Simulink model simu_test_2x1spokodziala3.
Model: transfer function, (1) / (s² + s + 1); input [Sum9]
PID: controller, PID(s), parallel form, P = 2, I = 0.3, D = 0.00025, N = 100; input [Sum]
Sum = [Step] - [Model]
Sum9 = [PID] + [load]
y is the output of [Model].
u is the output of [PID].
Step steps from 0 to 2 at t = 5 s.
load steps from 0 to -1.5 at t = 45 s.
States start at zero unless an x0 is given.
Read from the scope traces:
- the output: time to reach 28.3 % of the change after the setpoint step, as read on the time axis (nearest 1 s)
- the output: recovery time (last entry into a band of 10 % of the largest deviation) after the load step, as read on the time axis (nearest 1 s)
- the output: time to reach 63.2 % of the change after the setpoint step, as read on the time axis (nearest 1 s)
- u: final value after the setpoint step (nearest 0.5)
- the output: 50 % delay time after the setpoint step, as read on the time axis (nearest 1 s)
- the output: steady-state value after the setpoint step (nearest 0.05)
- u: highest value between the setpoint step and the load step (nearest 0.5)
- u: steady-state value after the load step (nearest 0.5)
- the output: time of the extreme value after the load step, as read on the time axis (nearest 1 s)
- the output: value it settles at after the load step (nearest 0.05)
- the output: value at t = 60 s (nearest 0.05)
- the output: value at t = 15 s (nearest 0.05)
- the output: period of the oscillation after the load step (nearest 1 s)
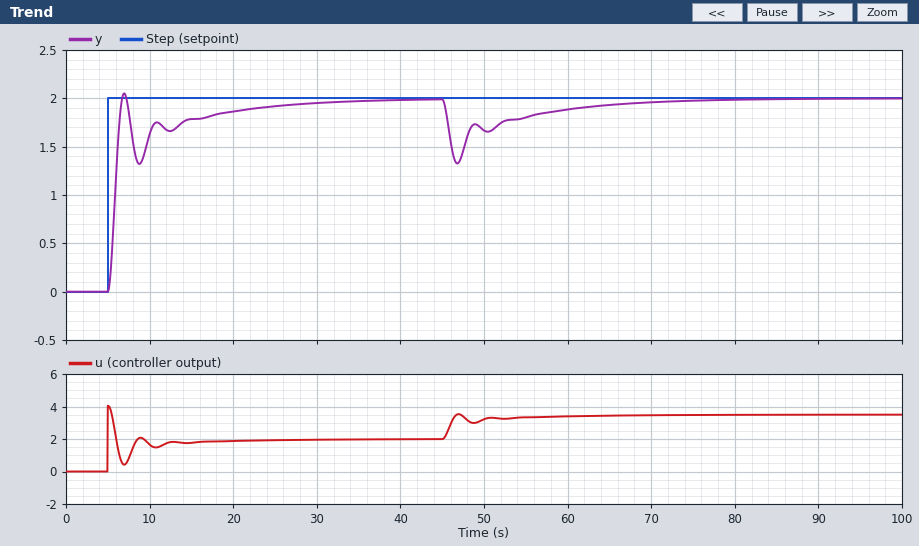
6 s
65 s
6 s
2.0
6 s
2.00
4.0
3.5
47 s
2.00
1.90
1.80
4 s
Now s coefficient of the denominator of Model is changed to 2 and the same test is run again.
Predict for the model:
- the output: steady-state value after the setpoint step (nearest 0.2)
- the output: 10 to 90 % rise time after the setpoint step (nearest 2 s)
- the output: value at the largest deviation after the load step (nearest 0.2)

2.0
10 s
1.4
